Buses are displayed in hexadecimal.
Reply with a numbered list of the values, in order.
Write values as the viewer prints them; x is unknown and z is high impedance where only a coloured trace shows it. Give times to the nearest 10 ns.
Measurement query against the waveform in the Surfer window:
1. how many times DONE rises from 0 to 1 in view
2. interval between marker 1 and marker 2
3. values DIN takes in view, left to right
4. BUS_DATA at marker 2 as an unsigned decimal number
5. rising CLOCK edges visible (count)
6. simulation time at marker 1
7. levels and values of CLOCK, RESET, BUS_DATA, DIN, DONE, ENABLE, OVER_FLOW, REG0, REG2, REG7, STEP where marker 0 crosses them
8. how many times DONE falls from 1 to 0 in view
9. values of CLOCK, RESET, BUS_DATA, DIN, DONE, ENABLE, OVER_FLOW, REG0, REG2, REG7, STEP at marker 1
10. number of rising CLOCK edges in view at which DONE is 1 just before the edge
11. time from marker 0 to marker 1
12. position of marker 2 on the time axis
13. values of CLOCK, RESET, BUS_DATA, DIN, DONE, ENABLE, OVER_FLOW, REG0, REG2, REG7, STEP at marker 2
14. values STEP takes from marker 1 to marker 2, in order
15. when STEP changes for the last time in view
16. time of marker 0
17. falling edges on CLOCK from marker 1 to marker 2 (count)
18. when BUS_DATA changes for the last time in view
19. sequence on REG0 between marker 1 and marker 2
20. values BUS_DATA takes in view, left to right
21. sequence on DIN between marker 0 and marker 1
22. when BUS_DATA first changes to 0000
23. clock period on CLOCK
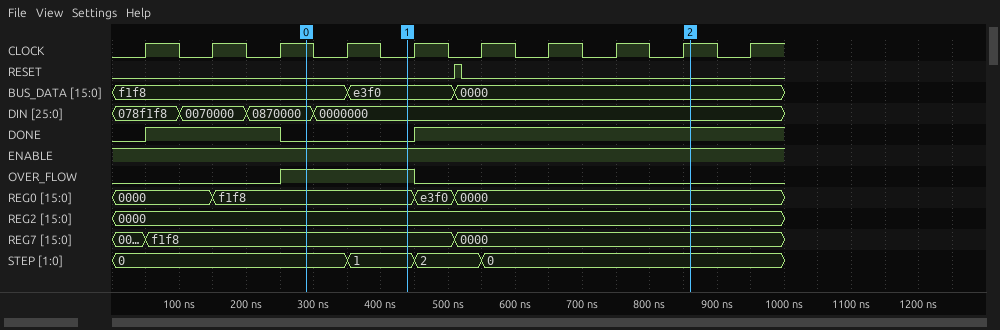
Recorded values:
1. 2
2. 420 ns
3. 078f1f8, 0070000, 0870000, 0000000
4. 0
5. 10
6. 440 ns
7. CLOCK=1, RESET=0, BUS_DATA=f1f8, DIN=0870000, DONE=0, ENABLE=1, OVER_FLOW=1, REG0=f1f8, REG2=0000, REG7=f1f8, STEP=0
8. 1
9. CLOCK=0, RESET=0, BUS_DATA=e3f0, DIN=0000000, DONE=0, ENABLE=1, OVER_FLOW=1, REG0=f1f8, REG2=0000, REG7=f1f8, STEP=1
10. 7
11. 150 ns
12. 860 ns
13. CLOCK=1, RESET=0, BUS_DATA=0000, DIN=0000000, DONE=1, ENABLE=1, OVER_FLOW=0, REG0=0000, REG2=0000, REG7=0000, STEP=0
14. 1, 2, 0
15. 550 ns
16. 290 ns
17. 4
18. 510 ns
19. f1f8, e3f0, 0000
20. f1f8, e3f0, 0000
21. 0870000, 0000000
22. 510 ns
23. 100 ns
